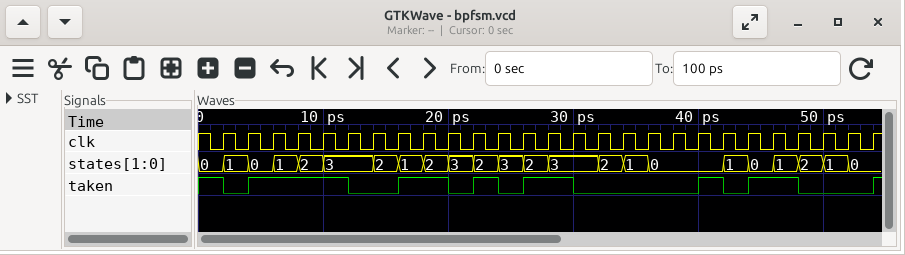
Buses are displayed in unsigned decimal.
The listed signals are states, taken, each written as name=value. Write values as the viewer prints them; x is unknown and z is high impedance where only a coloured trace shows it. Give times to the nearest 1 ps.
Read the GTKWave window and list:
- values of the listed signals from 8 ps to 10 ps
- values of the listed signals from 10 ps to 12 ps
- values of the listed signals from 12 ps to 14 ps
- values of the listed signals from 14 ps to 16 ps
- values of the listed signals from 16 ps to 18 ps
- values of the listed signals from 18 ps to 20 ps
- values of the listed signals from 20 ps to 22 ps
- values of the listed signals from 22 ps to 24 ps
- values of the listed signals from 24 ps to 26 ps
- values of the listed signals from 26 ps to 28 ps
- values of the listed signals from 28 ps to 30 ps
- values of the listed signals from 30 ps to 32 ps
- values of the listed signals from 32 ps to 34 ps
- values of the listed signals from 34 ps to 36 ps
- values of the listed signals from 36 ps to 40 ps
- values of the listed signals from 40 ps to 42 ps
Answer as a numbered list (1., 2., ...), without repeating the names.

1. states=2, taken=1
2. states=3, taken=1
3. states=3, taken=0
4. states=2, taken=0
5. states=1, taken=1
6. states=2, taken=1
7. states=3, taken=0
8. states=2, taken=1
9. states=3, taken=0
10. states=2, taken=1
11. states=3, taken=1
12. states=3, taken=0
13. states=2, taken=0
14. states=1, taken=0
15. states=0, taken=0
16. states=0, taken=1
